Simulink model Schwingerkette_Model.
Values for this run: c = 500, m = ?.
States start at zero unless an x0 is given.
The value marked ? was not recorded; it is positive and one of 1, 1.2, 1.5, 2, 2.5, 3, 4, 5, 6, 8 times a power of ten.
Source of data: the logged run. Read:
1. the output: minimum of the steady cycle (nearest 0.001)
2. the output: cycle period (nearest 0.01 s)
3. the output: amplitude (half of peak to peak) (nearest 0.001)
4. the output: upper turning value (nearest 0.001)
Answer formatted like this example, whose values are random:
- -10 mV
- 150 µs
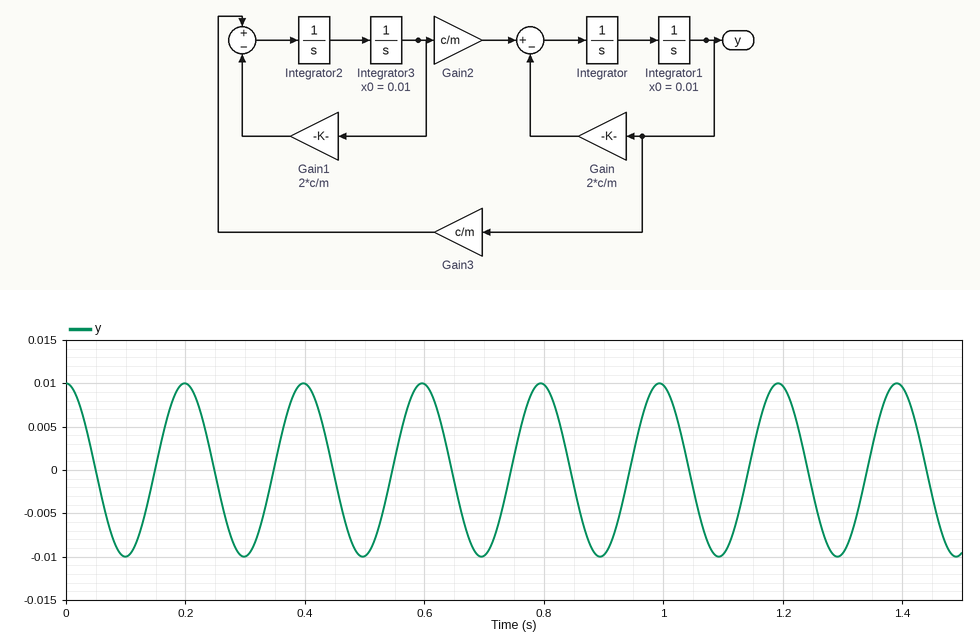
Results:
- -0.010
- 0.20 s
- 0.010
- 0.010
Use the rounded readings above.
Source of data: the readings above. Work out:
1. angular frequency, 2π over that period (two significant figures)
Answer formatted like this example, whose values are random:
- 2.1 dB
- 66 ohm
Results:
- 31 rad/s
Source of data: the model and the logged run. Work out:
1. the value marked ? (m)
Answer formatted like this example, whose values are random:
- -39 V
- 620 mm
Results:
- 0.5
